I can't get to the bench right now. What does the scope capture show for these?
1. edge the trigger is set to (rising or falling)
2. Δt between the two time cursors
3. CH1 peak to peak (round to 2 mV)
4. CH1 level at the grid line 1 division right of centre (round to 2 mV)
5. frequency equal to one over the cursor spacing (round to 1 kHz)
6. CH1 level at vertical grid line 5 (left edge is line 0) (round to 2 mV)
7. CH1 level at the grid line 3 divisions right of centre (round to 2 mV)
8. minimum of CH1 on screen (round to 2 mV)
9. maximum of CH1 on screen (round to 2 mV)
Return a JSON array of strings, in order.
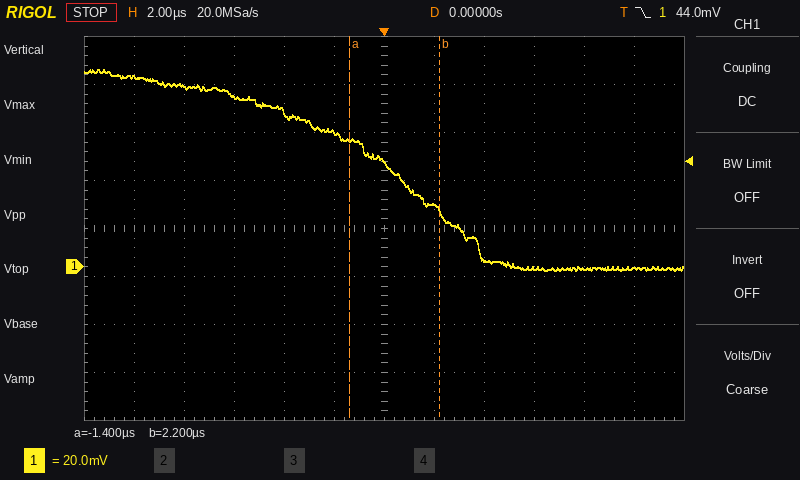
["falling", "3.6 µs", "84 mV", "26 mV", "278 kHz", "56 mV", "0 mV", "-2 mV", "82 mV"]
